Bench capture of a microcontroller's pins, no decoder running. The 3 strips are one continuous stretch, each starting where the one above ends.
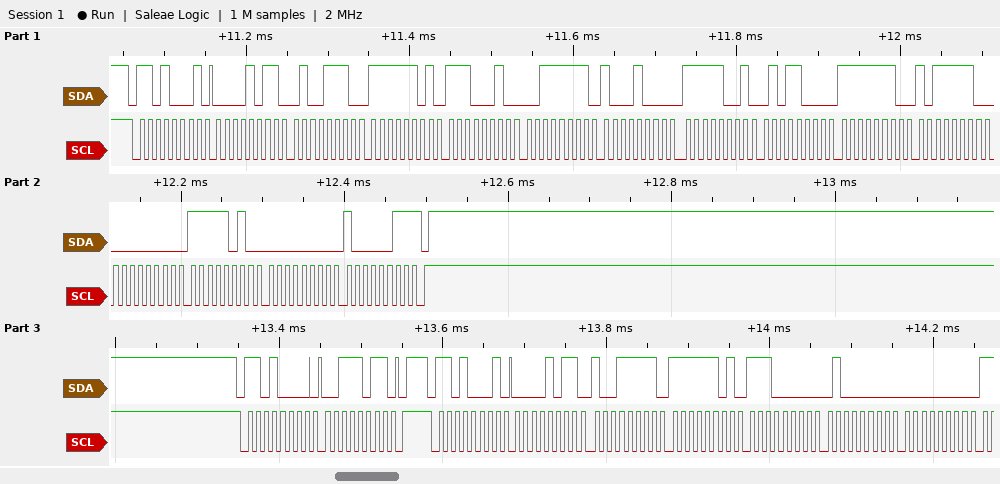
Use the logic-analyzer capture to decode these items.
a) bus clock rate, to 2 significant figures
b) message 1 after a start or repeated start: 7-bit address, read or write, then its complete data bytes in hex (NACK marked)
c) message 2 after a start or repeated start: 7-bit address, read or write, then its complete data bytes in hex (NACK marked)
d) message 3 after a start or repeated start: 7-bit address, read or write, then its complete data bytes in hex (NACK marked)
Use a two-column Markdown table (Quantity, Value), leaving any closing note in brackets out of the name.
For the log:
| Quantity | Value |
|---|---|
| bus clock rate, to 2 significant figures | 100 kHz |
| message 1 after a start or repeated start: 7-bit address, read or write, then its complete data bytes in hex | 0x68 read: 0B 4E FD E2 3F 88 F9 58 FE BE 00 FA 00 83 NACK |
| message 2 after a start or repeated start: 7-bit address, read or write, then its complete data bytes in hex | 0x68 write: 3B |
| message 3 after a start or repeated start: 7-bit address, read or write, then its complete data bytes in hex | 0x68 read: 0B 9F FD E0 40 00 |
